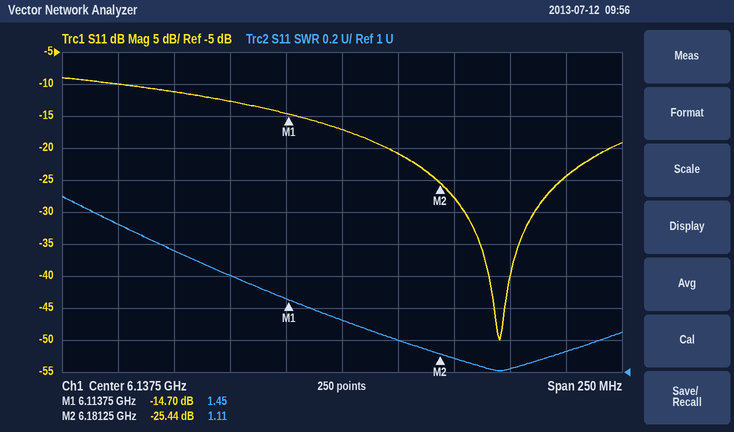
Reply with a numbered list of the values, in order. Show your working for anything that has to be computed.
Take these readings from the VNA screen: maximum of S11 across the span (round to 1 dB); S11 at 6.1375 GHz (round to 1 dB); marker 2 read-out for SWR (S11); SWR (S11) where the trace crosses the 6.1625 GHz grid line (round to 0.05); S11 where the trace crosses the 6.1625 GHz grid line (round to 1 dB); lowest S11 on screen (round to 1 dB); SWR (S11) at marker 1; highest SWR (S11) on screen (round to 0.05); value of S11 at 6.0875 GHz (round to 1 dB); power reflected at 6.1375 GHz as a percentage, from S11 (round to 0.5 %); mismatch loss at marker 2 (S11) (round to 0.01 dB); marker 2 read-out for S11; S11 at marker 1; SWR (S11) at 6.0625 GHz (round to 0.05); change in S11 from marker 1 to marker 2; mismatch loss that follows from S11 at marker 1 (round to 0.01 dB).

1. -9 dB
2. -17 dB
3. 1.11
4. 1.20
5. -21 dB
6. -50 dB
7. 1.45
8. 2.10
9. -13 dB
10. 10^(-17/10) ≈ 2.0 %
11. −10 log10(1 − 10^(-25.44/10)) ≈ 0.01 dB
12. -25.44 dB
13. -14.70 dB
14. 1.75
15. -25.44 − (-14.7) = -10.74 dB
16. −10 log10(1 − 10^(-14.7/10)) ≈ 0.15 dB
